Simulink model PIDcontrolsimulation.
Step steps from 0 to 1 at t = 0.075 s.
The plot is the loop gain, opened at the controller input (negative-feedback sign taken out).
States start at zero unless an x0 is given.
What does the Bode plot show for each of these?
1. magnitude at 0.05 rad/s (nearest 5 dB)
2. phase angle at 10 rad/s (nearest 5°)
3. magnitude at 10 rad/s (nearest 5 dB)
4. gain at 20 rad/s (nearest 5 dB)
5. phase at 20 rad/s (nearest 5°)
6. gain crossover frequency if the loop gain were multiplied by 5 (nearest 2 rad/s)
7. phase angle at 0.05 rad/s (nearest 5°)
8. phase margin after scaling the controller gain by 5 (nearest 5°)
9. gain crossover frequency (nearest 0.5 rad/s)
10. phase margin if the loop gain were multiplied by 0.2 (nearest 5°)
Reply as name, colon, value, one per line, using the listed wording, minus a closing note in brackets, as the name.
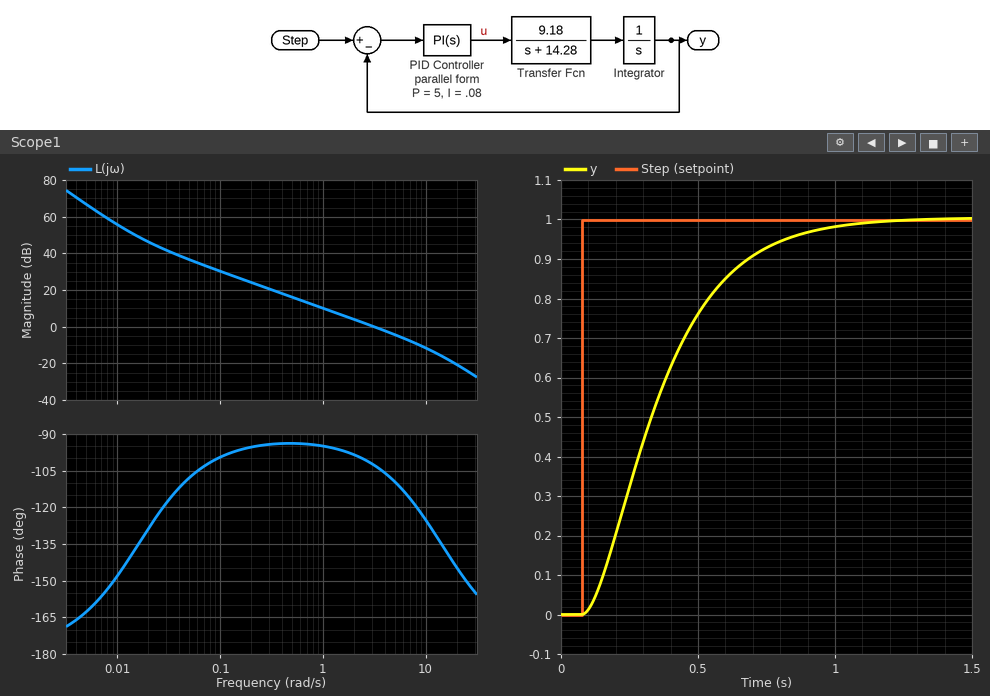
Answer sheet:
magnitude at 0.05 rad/s: 35 dB
phase angle at 10 rad/s: -125°
magnitude at 10 rad/s: -10 dB
gain at 20 rad/s: -20 dB
phase at 20 rad/s: -145°
gain crossover frequency if the loop gain were multiplied by 5: 12 rad/s
phase angle at 0.05 rad/s: -110°
phase margin after scaling the controller gain by 5: 50°
gain crossover frequency: 3.0 rad/s
phase margin if the loop gain were multiplied by 0.2: 85°
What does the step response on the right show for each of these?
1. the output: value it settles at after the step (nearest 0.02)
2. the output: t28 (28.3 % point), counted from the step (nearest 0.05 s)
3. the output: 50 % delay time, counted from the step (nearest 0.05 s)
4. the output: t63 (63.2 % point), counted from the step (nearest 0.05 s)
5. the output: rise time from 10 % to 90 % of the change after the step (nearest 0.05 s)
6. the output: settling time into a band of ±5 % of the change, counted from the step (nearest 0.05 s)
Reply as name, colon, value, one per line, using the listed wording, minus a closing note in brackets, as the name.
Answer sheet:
the output: value it settles at after the step: 1.00
the output: t28 (28.3 % point), counted from the step: 0.15 s
the output: 50 % delay time, counted from the step: 0.25 s
the output: t63 (63.2 % point), counted from the step: 0.35 s
the output: rise time from 10 % to 90 % of the change after the step: 0.55 s
the output: settling time into a band of ±5 % of the change, counted from the step: 0.75 s
